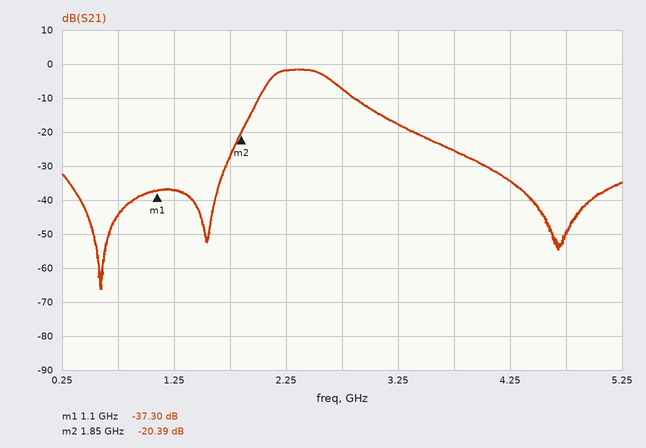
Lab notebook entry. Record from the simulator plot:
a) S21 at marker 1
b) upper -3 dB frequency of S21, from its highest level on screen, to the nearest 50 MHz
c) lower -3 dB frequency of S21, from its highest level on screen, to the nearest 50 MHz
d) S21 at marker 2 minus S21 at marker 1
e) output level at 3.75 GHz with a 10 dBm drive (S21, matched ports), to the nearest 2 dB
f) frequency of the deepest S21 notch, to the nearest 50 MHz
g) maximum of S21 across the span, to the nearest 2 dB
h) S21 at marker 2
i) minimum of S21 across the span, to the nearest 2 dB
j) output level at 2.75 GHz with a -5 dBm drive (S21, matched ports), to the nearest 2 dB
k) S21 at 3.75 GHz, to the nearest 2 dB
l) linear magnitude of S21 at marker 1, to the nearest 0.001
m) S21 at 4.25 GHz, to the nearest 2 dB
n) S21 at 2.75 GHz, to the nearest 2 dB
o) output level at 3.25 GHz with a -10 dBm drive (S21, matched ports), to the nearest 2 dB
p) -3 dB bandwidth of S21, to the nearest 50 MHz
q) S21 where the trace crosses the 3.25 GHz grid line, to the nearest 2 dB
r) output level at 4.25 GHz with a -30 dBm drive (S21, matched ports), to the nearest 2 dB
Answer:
-37.30 dB
2.65 GHz
2.10 GHz
16.91 dB
-16 dBm
600 MHz
-2 dB
-20.39 dB
-66 dB
-12 dBm
-26 dB
0.014
-34 dB
-8 dB
-28 dBm
550 MHz
-18 dB
-64 dBm
